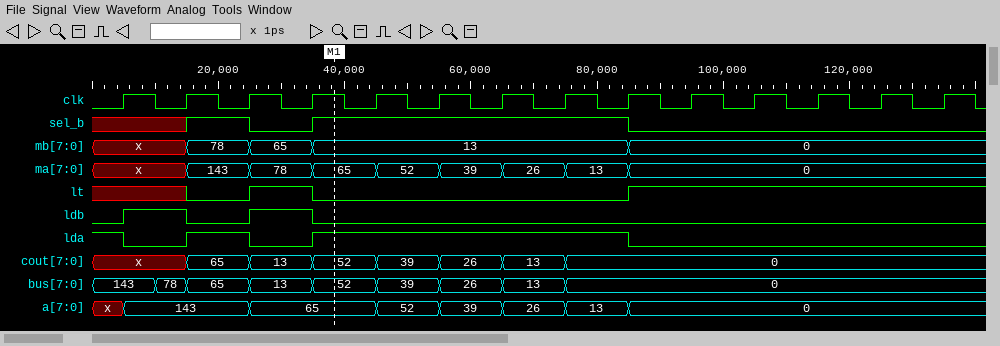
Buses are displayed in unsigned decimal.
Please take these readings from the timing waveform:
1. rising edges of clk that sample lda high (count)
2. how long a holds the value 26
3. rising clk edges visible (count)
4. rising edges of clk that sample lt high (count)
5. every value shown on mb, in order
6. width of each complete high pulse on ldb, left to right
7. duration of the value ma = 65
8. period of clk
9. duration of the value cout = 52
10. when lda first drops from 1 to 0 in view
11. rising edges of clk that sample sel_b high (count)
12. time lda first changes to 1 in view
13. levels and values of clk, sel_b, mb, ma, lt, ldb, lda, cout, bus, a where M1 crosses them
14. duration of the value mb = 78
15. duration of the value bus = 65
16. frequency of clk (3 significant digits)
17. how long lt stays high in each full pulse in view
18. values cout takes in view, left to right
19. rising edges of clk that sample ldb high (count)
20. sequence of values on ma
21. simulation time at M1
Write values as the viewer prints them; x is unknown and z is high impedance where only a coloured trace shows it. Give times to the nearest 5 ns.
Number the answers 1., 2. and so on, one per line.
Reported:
1. 7
2. 10 ns
3. 14
4. 6
5. x, 78, 65, 13, 0
6. 10 ns, 10 ns
7. 10 ns
8. 10 ns
9. 10 ns
10. 5 ns
11. 6
12. 15 ns
13. clk=1, sel_b=1, mb=13, ma=65, lt=0, ldb=0, lda=1, cout=52, bus=52, a=65
14. 10 ns
15. 10 ns
16. 100 MHz
17. 10 ns
18. x, 65, 13, 52, 39, 26, 13, 0
19. 2
20. x, 143, 78, 65, 52, 39, 26, 13, 0
21. 40 ns
